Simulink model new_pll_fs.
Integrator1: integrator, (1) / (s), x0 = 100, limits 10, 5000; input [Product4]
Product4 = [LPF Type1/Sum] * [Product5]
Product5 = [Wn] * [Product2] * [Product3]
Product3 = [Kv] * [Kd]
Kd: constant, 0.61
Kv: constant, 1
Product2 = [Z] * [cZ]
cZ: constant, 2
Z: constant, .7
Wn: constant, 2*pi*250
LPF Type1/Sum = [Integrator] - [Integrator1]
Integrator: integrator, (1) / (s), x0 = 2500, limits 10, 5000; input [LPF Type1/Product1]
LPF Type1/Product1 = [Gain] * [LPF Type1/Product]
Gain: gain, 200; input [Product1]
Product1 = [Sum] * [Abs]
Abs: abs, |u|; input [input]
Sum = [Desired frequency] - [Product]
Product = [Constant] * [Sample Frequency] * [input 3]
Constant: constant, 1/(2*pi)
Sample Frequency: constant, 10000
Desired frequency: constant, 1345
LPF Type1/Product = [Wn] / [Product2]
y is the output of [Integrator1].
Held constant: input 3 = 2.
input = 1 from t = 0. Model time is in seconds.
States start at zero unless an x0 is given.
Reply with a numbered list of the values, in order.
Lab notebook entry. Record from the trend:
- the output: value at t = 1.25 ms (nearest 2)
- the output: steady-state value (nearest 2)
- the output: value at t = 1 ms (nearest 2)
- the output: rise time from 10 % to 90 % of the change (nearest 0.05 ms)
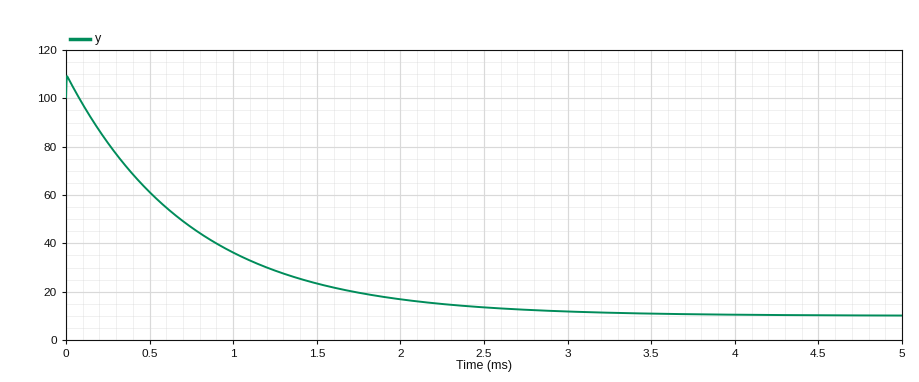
1. 28
2. 10
3. 36
4. 1.65 ms
